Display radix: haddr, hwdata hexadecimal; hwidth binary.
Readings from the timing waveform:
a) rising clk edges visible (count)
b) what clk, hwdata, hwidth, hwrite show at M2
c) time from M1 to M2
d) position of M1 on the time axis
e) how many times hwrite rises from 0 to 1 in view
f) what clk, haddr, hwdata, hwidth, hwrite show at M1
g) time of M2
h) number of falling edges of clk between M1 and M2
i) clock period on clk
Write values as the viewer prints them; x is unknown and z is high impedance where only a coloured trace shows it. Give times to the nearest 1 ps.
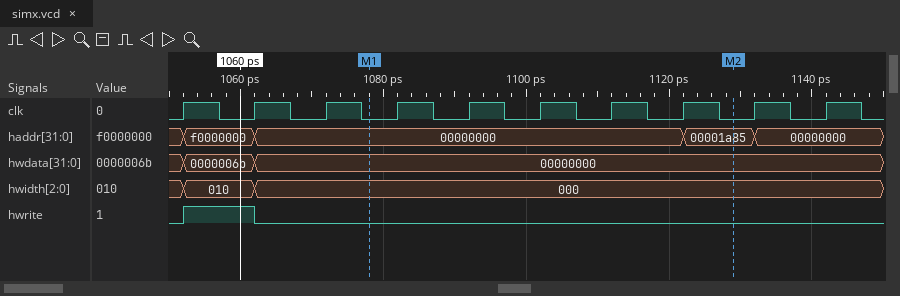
10
clk=0, hwdata=00000000, hwidth=000, hwrite=0
51 ps
1078 ps
1
clk=0, haddr=00000000, hwdata=00000000, hwidth=000, hwrite=0
1129 ps
5
10 ps
